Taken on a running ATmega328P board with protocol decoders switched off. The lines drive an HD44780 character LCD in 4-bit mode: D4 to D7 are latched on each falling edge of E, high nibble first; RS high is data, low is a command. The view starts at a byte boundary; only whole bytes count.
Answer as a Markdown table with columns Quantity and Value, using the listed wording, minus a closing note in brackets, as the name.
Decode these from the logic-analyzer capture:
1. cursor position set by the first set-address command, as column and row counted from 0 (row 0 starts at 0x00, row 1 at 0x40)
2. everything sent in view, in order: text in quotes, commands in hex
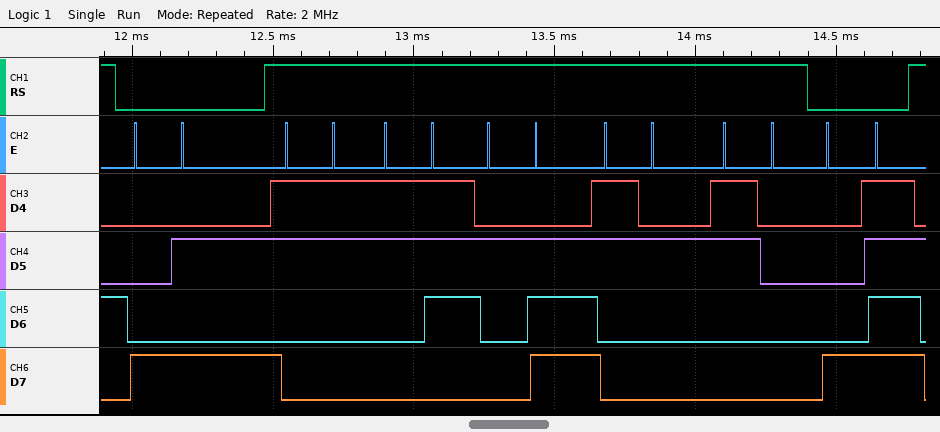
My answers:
| Quantity | Value |
|---|---|
| cursor position set by the first set-address command, as column and row counted from 0 | column 10, row 0 |
| everything sent in view, in order: text in quotes, commands in hex | 0x8A "37.20" 0x8F |
